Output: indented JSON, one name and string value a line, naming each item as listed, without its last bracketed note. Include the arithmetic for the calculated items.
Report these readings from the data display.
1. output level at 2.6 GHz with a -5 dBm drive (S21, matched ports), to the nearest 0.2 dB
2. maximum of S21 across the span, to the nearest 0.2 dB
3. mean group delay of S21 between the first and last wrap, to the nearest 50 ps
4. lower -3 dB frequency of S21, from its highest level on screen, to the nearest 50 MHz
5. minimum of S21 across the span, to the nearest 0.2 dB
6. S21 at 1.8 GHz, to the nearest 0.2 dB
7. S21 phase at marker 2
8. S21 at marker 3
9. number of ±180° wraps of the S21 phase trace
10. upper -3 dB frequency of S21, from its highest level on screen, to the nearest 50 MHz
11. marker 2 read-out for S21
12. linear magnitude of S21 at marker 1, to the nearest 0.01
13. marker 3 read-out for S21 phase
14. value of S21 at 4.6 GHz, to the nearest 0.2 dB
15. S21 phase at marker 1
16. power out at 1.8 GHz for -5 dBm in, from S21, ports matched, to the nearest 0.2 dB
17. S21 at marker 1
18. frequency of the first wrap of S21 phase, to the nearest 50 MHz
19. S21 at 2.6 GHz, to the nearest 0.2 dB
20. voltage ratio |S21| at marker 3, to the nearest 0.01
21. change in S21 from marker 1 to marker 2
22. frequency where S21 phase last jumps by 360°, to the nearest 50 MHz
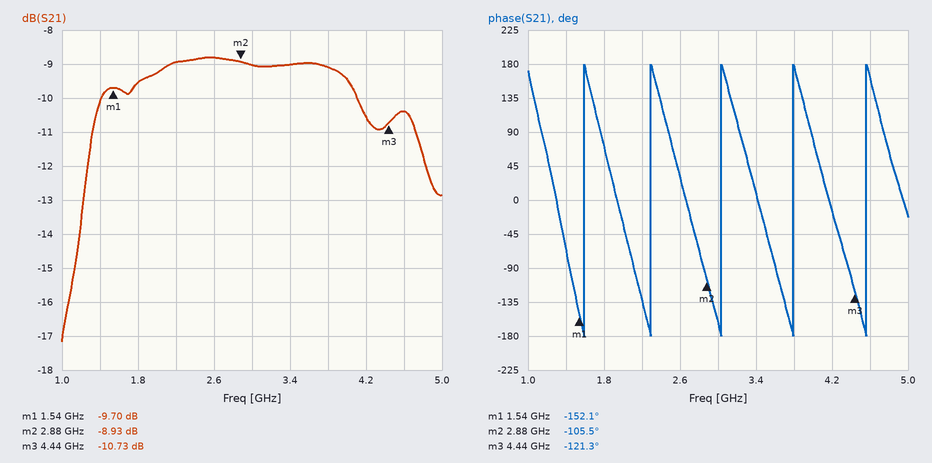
{
  "output level at 2.6 GHz with a -5 dBm drive (S21, matched ports), to the nearest 0.2 dB": "-5 dBm + (-8.8 dB) = -13.8 dBm",
  "maximum of S21 across the span, to the nearest 0.2 dB": "-8.8 dB",
  "mean group delay of S21 between the first and last wrap, to the nearest 50 ps": "4 cycles / (4.55 GHz − 1.60 GHz) ≈ 1.36 ns, so 1.35 ns to the nearest 50 ps",
  "lower -3 dB frequency of S21, from its highest level on screen, to the nearest 50 MHz": "1.30 GHz",
  "minimum of S21 across the span, to the nearest 0.2 dB": "-17.2 dB",
  "S21 at 1.8 GHz, to the nearest 0.2 dB": "-9.6 dB",
  "S21 phase at marker 2": "-105.5°",
  "S21 at marker 3": "-10.73 dB",
  "number of ±180° wraps of the S21 phase trace": "5",
  "upper -3 dB frequency of S21, from its highest level on screen, to the nearest 50 MHz": "4.80 GHz",
  "marker 2 read-out for S21": "-8.93 dB",
  "linear magnitude of S21 at marker 1, to the nearest 0.01": "10^(-9.7/20) ≈ 0.33",
  "marker 3 read-out for S21 phase": "-121.3°",
  "value of S21 at 4.6 GHz, to the nearest 0.2 dB": "-10.4 dB",
  "S21 phase at marker 1": "-152.1°",
  "power out at 1.8 GHz for -5 dBm in, from S21, ports matched, to the nearest 0.2 dB": "-5 dBm + (-9.6 dB) = -14.6 dBm",
  "S21 at marker 1": "-9.70 dB",
  "frequency of the first wrap of S21 phase, to the nearest 50 MHz": "1.60 GHz",
  "S21 at 2.6 GHz, to the nearest 0.2 dB": "-8.8 dB",
  "voltage ratio |S21| at marker 3, to the nearest 0.01": "10^(-10.73/20) ≈ 0.29",
  "change in S21 from marker 1 to marker 2": "-8.93 − (-9.7) = 0.77 dB",
  "frequency where S21 phase last jumps by 360°, to the nearest 50 MHz": "4.55 GHz"
}
